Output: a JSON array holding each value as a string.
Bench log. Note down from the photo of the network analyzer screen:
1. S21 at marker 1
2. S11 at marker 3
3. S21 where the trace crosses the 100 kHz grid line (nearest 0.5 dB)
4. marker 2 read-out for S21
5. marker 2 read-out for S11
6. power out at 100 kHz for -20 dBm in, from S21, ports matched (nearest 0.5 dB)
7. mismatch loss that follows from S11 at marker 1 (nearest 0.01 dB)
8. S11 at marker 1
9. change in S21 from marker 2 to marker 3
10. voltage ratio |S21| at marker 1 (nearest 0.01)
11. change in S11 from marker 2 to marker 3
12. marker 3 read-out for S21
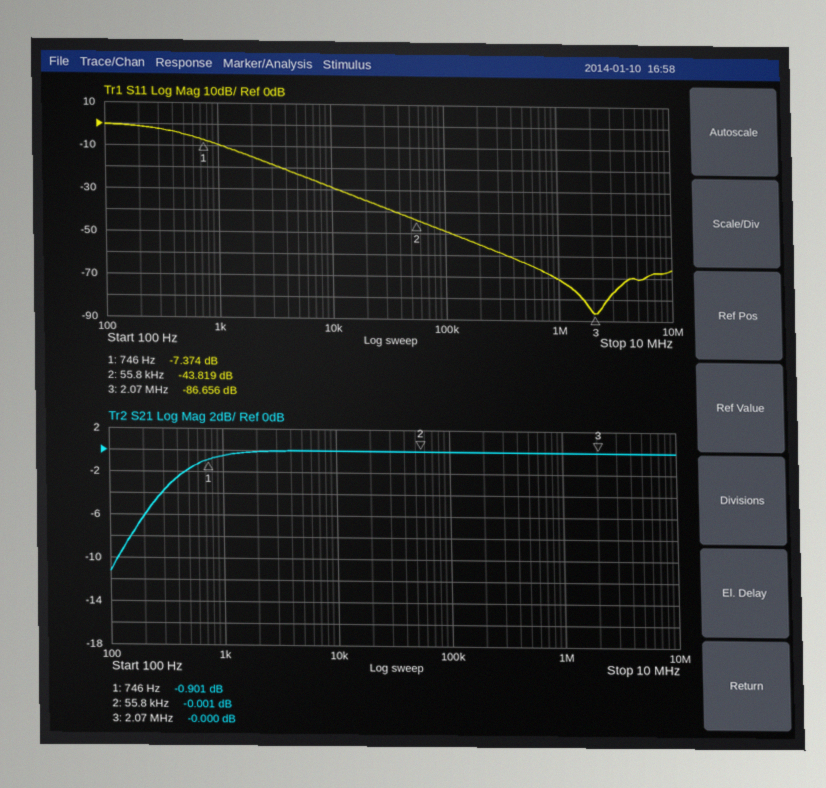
["-0.901 dB", "-86.656 dB", "0.0 dB", "-0.001 dB", "-43.819 dB", "-20.0 dBm", "0.88 dB", "-7.374 dB", "0.001 dB", "0.90", "-42.837 dB", "-0.000 dB"]
